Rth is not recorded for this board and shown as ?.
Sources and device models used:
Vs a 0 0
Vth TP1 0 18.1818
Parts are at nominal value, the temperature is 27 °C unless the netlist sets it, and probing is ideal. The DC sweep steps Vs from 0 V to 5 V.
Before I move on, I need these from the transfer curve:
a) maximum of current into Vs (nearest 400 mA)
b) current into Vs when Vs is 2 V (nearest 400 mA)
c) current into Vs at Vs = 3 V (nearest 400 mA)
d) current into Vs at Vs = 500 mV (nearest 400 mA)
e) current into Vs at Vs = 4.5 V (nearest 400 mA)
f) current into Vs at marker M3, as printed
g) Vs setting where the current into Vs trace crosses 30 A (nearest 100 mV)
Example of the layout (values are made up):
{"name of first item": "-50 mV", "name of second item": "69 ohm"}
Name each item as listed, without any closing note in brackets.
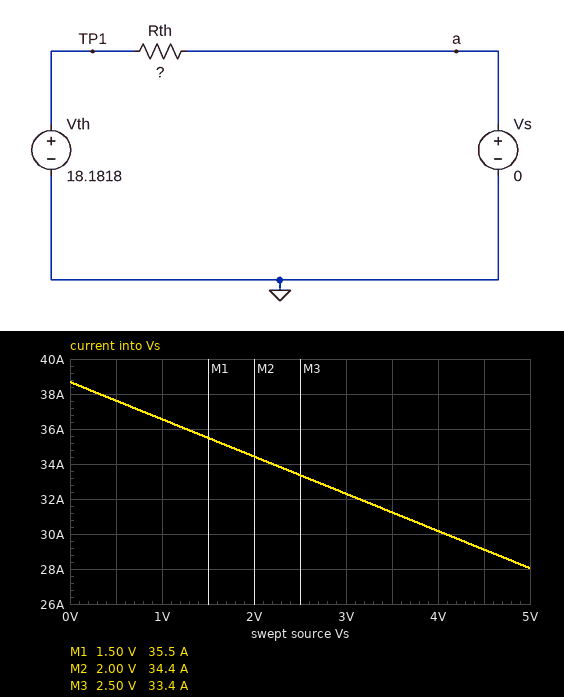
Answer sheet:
{"maximum of current into Vs": "38.8 A", "current into Vs when Vs is 2 V": "34.4 A", "current into Vs at Vs = 3 V": "32.4 A", "current into Vs at Vs = 500 mV": "37.6 A", "current into Vs at Vs = 4.5 V": "29.2 A", "current into Vs at marker M3, as printed": "33.4 A", "Vs setting where the current into Vs trace crosses 30 A": "4.1 V"}
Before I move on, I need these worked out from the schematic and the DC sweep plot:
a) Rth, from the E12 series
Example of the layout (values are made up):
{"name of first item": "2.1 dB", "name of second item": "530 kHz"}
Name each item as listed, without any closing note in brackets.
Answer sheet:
{"Rth, from the E12 series": "0.47 Ω"}
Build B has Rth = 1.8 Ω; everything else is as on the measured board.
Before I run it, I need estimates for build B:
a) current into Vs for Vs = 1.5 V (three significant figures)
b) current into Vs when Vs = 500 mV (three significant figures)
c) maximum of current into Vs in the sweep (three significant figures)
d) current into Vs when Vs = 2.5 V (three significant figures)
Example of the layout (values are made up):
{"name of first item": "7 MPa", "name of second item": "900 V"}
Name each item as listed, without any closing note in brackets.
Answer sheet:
{"current into Vs for Vs = 1.5 V": "9.27 A", "current into Vs when Vs = 500 mV": "9.82 A", "maximum of current into Vs in the sweep": "10.1 A", "current into Vs when Vs = 2.5 V": "8.71 A"}
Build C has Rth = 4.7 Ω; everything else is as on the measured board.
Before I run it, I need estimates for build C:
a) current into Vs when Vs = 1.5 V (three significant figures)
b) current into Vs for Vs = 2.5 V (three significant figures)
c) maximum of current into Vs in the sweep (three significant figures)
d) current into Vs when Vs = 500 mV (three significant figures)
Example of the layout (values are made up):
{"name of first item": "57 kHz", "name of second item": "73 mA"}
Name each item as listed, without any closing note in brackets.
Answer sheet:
{"current into Vs when Vs = 1.5 V": "3.55 A", "current into Vs for Vs = 2.5 V": "3.34 A", "maximum of current into Vs in the sweep": "3.87 A", "current into Vs when Vs = 500 mV": "3.76 A"}
